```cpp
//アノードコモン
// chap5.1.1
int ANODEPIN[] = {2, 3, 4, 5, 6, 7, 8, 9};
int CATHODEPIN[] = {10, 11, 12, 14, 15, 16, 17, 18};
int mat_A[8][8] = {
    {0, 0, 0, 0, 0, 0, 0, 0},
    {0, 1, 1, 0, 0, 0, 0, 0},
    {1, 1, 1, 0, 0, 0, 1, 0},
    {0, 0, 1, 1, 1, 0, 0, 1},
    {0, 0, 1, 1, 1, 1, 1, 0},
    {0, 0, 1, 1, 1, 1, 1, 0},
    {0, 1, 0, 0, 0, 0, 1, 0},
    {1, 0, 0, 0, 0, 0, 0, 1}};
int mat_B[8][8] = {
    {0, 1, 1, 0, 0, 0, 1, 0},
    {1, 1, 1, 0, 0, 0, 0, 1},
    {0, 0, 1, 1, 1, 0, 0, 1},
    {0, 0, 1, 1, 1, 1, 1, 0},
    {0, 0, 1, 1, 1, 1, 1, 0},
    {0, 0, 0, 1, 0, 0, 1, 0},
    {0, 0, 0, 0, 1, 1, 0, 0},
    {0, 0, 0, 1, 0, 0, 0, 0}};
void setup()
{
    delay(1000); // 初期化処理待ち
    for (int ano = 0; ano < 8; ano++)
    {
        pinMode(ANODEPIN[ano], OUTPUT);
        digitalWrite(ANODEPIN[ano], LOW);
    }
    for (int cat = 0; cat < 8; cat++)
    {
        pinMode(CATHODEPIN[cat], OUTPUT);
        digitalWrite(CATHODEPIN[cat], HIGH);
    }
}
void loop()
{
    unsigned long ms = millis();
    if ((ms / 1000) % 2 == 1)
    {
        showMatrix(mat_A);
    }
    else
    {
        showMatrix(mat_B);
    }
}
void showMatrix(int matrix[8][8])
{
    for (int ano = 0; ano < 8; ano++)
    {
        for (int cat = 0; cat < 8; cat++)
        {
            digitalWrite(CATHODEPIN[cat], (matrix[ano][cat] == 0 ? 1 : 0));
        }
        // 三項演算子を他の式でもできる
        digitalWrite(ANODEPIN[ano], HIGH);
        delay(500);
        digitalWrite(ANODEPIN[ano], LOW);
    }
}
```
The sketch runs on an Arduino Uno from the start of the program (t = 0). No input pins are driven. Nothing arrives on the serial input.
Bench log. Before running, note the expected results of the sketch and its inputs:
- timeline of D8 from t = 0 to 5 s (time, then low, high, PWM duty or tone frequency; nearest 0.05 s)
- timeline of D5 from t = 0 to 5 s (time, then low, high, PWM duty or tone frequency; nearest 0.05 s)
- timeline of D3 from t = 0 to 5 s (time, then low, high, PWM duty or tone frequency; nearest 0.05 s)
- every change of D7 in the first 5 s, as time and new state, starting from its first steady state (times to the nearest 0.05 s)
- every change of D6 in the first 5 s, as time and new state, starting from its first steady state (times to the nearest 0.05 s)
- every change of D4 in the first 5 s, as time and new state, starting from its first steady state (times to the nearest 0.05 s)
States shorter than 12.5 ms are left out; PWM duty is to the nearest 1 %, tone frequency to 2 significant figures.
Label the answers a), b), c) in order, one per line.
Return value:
a) 1 s low; 4 s high; 4.5 s low
b) 1 s low; 2.5 s high; 3 s low
c) 1 s low; 1.5 s high; 2 s low
d) 1 s low; 3.5 s high; 4 s low
e) 1 s low; 3 s high; 3.5 s low
f) 1 s low; 2 s high; 2.5 s low
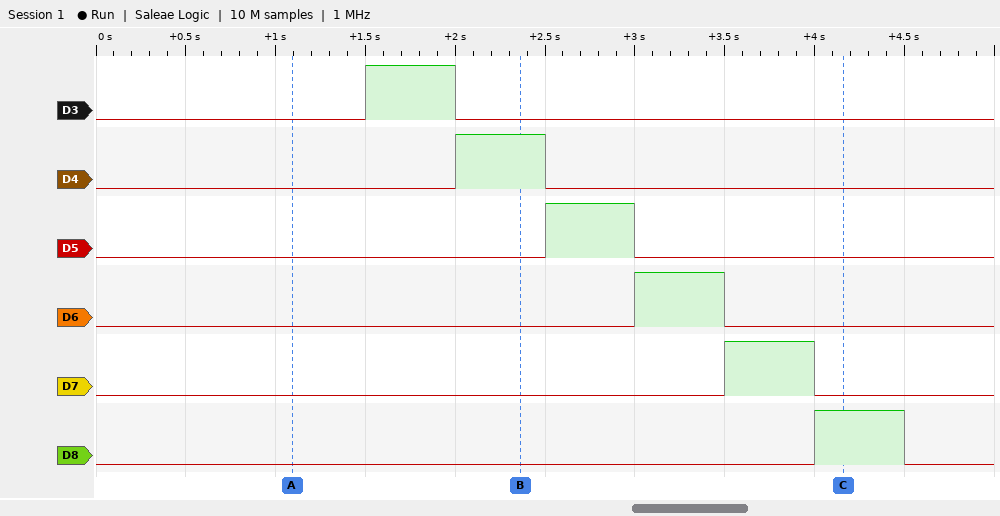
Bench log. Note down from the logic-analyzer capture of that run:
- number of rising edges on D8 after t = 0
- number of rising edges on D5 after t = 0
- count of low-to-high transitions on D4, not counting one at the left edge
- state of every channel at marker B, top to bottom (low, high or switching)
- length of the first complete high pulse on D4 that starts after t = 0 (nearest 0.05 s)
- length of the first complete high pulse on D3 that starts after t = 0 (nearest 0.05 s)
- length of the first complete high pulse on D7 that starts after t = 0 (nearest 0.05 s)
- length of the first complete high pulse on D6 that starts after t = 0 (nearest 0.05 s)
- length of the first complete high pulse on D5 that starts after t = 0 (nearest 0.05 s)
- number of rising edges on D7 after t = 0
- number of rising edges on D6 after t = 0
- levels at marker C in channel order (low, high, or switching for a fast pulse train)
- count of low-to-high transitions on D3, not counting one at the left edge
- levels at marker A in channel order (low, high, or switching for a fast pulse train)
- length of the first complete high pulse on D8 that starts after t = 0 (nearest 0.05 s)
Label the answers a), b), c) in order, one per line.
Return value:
a) 1
b) 1
c) 1
d) D3 low, D4 high, D5 low, D6 low, D7 low, D8 low
e) 0.50 s
f) 0.50 s
g) 0.50 s
h) 0.50 s
i) 0.50 s
j) 1
k) 1
l) D3 low, D4 low, D5 low, D6 low, D7 low, D8 high
m) 1
n) D3 low, D4 low, D5 low, D6 low, D7 low, D8 low
o) 0.50 s
